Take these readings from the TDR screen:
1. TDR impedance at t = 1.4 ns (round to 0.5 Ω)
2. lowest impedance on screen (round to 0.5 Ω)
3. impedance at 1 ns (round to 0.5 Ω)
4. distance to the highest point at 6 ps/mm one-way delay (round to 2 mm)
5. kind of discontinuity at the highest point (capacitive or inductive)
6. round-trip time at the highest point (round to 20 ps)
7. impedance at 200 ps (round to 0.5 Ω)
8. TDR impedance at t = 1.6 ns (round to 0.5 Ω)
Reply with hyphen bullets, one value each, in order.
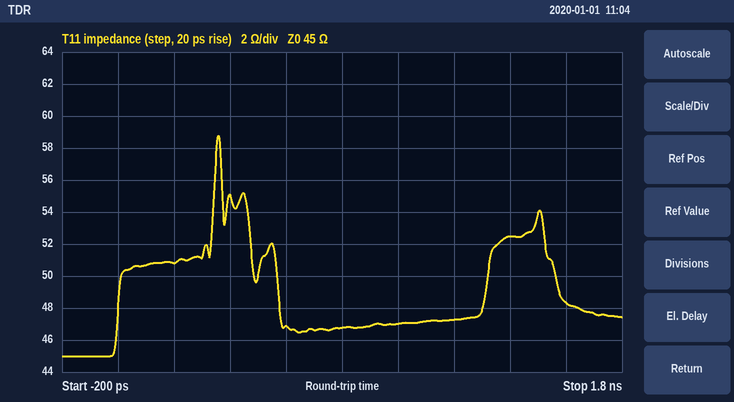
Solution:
- 52.5 Ω
- 45.0 Ω
- 47.0 Ω
- 30 mm
- inductive
- 360 ps
- 51.0 Ω
- 48.5 Ω
